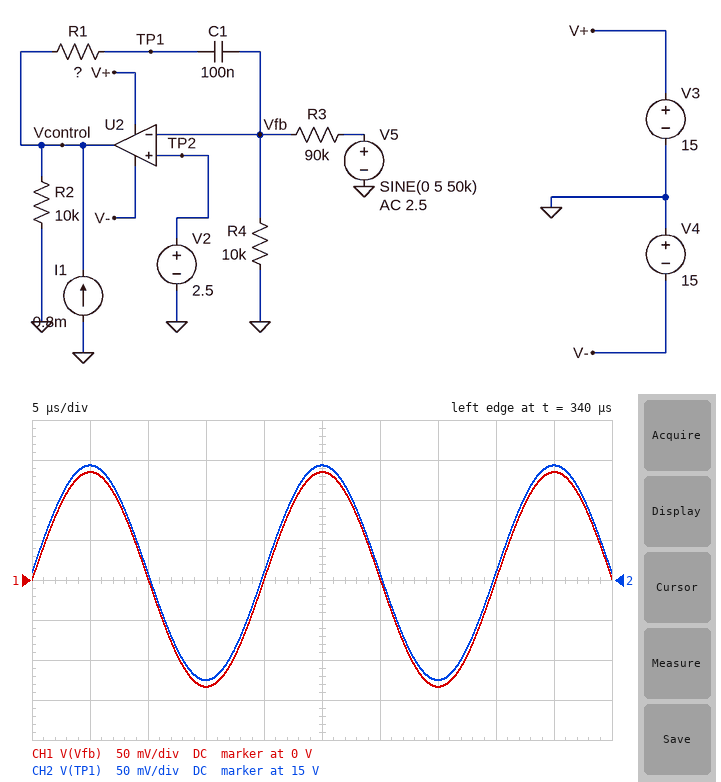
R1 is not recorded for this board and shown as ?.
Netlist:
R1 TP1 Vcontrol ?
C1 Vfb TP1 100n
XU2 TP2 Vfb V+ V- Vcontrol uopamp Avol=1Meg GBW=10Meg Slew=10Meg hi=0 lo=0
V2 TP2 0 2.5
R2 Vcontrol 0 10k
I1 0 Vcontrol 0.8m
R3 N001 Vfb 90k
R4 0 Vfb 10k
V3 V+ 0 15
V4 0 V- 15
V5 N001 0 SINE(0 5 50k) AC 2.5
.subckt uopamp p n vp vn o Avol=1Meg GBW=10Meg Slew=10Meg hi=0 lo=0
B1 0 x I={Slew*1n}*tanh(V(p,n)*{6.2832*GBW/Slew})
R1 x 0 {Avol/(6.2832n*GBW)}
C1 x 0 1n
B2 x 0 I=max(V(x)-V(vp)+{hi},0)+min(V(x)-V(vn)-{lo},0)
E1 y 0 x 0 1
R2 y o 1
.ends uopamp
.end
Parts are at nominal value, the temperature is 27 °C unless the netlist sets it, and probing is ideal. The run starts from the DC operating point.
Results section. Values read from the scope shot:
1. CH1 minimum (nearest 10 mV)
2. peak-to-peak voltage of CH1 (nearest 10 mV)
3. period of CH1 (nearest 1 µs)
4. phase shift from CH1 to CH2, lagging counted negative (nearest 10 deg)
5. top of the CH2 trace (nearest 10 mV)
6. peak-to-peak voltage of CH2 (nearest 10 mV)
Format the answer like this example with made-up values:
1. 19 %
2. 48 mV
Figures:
1. -130 mV
2. 270 mV
3. 20 µs
4. 0 deg
5. 15.14 V
6. 270 mV
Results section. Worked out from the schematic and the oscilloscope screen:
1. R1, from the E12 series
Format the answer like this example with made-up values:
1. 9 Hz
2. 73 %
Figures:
1. 3.3 kΩ
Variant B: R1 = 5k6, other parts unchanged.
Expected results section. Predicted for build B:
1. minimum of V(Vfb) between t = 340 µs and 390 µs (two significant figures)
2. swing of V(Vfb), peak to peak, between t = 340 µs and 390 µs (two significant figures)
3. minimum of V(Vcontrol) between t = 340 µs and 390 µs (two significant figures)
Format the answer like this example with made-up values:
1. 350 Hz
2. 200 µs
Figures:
1. -190 mV
2. 380 mV
3. 15 V
